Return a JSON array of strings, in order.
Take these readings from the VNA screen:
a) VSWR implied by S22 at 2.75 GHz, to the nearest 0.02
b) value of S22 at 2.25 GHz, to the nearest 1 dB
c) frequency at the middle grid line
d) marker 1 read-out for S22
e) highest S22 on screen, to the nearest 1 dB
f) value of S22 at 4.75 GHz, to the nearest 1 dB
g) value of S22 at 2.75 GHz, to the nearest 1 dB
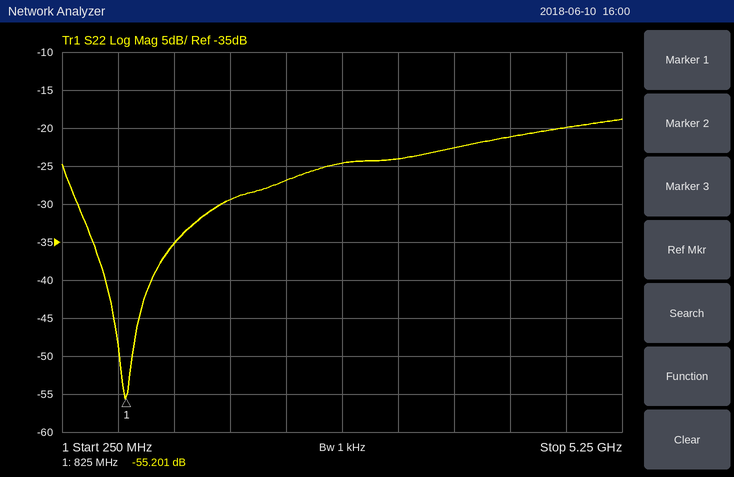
["1.12", "-27 dB", "2.75 GHz", "-55.201 dB", "-19 dB", "-20 dB", "-25 dB"]
